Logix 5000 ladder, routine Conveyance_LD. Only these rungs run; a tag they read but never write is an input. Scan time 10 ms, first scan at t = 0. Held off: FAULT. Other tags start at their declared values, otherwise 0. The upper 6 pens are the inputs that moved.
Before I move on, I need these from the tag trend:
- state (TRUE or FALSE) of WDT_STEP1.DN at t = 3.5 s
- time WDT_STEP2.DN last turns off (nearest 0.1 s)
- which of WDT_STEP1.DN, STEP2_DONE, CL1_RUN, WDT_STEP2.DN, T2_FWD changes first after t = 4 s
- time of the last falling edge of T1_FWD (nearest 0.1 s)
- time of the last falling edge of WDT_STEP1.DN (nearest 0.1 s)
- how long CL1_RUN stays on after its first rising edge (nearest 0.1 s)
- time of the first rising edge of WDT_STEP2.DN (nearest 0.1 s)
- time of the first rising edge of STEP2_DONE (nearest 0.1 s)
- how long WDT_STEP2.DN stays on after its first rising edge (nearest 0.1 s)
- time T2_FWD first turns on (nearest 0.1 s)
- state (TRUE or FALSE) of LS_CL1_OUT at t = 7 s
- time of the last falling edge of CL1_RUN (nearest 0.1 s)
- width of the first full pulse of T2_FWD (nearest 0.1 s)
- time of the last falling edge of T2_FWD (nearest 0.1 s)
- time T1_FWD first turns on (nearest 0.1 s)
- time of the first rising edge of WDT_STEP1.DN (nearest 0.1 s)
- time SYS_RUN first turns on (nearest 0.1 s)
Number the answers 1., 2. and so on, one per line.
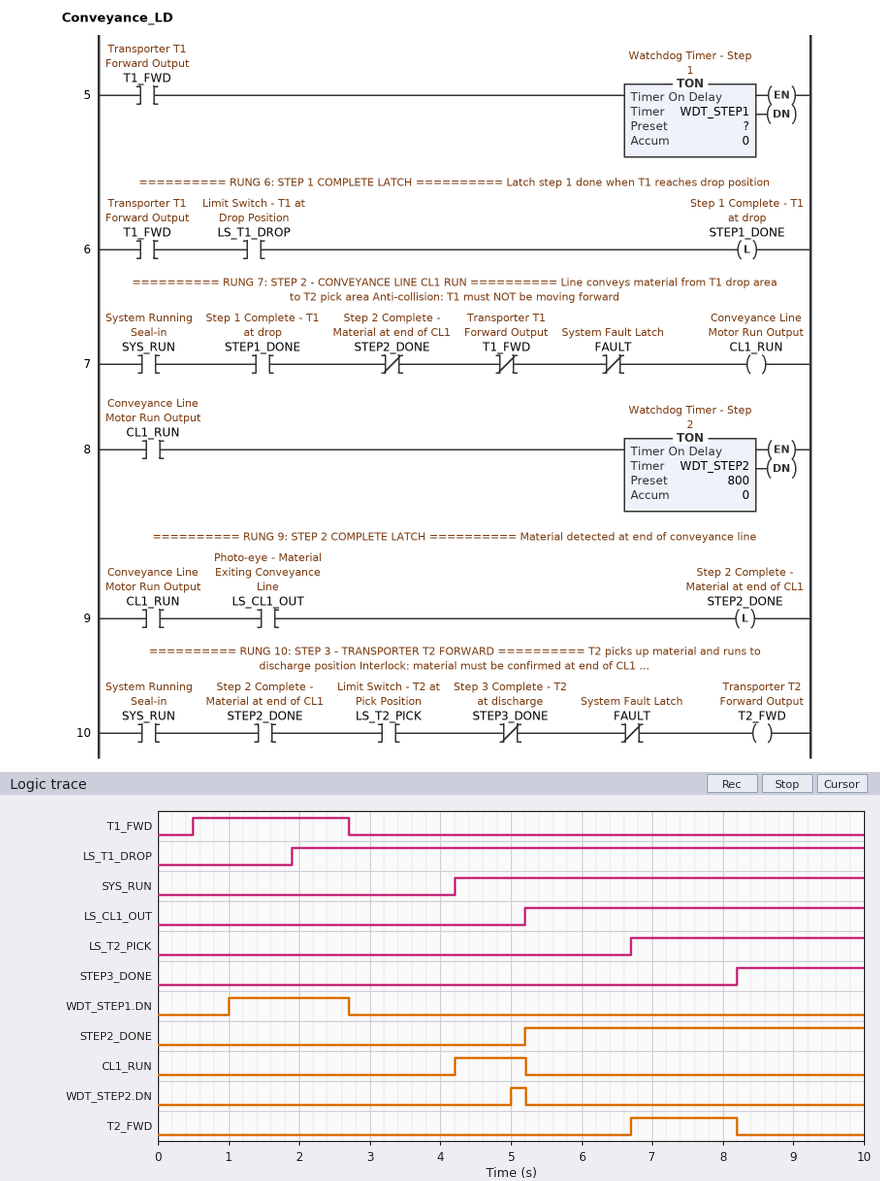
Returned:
1. FALSE
2. 5.2 s
3. CL1_RUN
4. 2.7 s
5. 2.7 s
6. 1.0 s
7. 5.0 s
8. 5.2 s
9. 0.2 s
10. 6.7 s
11. TRUE
12. 5.2 s
13. 1.5 s
14. 8.2 s
15. 0.5 s
16. 1.0 s
17. 4.2 s
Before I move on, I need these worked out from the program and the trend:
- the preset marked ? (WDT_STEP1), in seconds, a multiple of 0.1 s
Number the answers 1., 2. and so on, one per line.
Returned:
1. 0.5 s
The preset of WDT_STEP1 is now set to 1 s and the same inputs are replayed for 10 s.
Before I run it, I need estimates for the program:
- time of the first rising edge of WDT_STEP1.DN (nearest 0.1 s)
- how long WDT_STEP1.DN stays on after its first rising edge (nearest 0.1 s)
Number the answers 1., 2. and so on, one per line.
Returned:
1. 1.5 s
2. 1.2 s
